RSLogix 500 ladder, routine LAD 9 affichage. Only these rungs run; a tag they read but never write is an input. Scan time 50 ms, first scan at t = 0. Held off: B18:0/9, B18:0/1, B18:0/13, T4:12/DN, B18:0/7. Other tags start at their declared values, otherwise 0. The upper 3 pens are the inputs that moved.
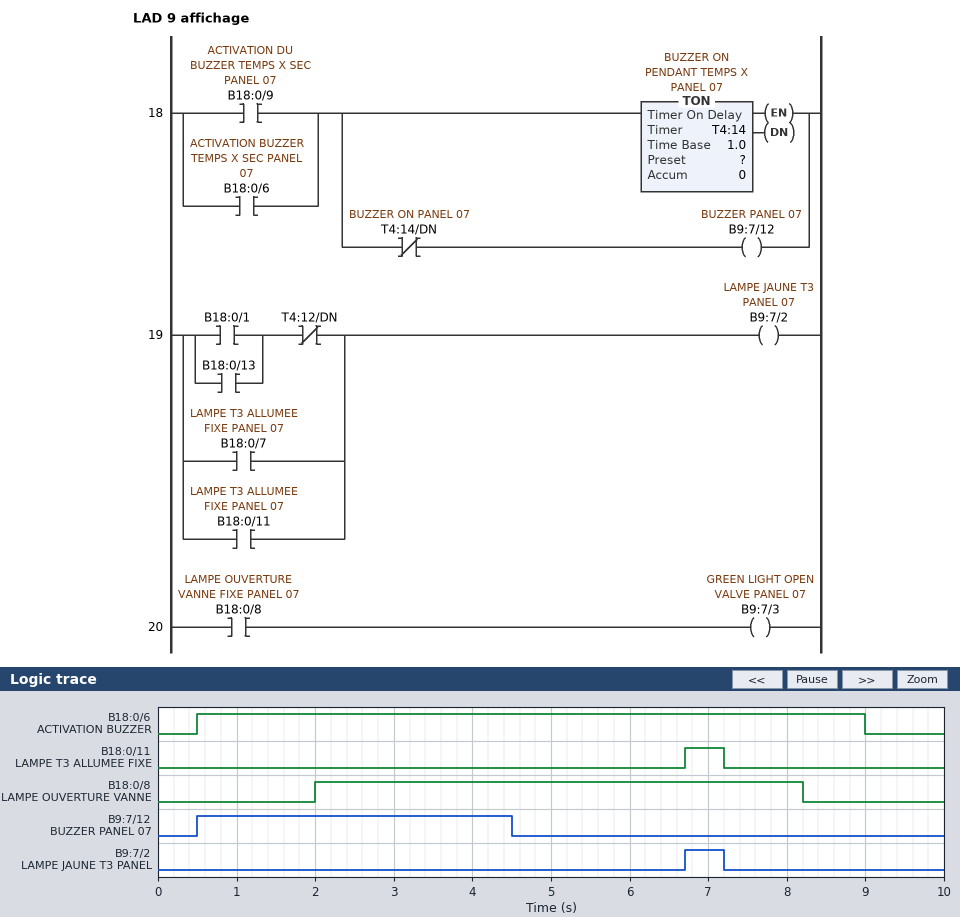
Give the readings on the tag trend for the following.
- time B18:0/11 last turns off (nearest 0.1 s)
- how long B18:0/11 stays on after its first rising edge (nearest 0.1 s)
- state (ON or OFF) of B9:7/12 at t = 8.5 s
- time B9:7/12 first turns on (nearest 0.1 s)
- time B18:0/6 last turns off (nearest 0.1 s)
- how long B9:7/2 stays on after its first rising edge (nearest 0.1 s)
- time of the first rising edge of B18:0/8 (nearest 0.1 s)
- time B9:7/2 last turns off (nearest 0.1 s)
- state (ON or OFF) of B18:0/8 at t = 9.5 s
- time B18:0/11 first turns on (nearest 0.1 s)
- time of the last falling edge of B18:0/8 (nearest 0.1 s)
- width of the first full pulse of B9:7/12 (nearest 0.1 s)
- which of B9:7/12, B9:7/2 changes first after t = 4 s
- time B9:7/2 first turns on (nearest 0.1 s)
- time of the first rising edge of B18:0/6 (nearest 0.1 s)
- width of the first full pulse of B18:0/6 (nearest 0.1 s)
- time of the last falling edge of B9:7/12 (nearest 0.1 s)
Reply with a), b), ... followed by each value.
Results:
a) 7.2 s
b) 0.5 s
c) OFF
d) 0.5 s
e) 9.0 s
f) 0.5 s
g) 2.0 s
h) 7.2 s
i) OFF
j) 6.7 s
k) 8.2 s
l) 4.0 s
m) B9:7/12
n) 6.7 s
o) 0.5 s
p) 8.5 s
q) 4.5 s
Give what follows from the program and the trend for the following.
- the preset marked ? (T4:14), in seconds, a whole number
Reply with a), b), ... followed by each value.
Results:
a) 4 s
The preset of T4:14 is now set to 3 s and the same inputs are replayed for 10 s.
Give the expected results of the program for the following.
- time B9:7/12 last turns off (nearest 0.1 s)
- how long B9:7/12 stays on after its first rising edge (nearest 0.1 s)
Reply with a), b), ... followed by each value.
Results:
a) 3.5 s
b) 3.0 s
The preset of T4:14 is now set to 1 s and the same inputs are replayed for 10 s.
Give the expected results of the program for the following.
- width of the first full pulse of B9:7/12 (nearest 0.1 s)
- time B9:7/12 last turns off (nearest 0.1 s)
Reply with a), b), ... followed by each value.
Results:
a) 1.0 s
b) 1.5 s
